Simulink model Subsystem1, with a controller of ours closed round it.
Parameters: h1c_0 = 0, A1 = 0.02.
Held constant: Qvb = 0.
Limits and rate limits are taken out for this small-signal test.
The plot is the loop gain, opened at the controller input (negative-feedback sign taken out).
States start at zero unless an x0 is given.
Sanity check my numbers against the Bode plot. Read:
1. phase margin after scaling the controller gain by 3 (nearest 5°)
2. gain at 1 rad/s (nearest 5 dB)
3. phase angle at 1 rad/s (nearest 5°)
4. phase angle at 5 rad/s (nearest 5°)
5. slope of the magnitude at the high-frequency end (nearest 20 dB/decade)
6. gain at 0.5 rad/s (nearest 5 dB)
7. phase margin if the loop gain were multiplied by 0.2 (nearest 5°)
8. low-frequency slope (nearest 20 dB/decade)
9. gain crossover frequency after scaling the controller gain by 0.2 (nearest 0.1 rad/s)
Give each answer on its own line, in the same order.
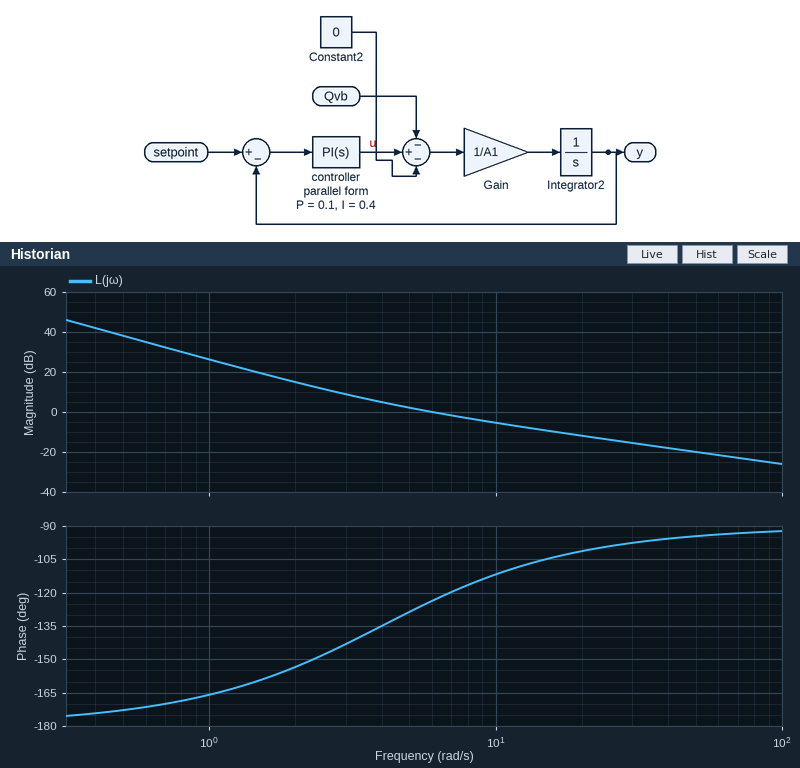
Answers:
75°
25 dB
-165°
-130°
-20 dB/decade
40 dB
30°
-40 dB/decade
2.1 rad/s
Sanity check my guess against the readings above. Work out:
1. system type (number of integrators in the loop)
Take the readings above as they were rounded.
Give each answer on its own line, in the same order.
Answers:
2
